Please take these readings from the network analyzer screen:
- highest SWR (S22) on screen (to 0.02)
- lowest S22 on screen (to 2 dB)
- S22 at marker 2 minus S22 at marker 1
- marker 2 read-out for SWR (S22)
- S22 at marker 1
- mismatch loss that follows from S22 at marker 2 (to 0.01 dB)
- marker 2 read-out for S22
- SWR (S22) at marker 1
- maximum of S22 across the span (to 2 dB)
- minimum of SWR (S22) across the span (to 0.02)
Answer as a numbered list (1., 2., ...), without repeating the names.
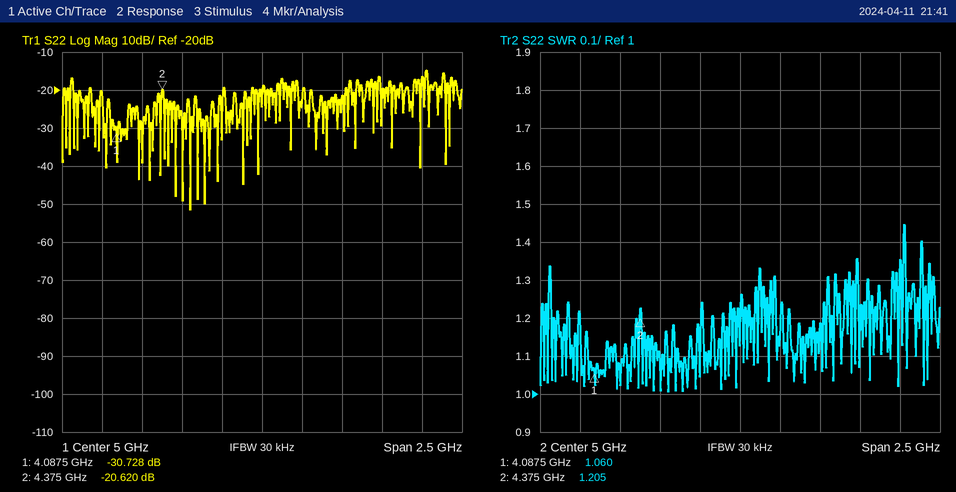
1. 1.44
2. -52 dB
3. 10.108 dB
4. 1.205
5. -30.728 dB
6. 0.04 dB
7. -20.620 dB
8. 1.060
9. -14 dB
10. 1.00
